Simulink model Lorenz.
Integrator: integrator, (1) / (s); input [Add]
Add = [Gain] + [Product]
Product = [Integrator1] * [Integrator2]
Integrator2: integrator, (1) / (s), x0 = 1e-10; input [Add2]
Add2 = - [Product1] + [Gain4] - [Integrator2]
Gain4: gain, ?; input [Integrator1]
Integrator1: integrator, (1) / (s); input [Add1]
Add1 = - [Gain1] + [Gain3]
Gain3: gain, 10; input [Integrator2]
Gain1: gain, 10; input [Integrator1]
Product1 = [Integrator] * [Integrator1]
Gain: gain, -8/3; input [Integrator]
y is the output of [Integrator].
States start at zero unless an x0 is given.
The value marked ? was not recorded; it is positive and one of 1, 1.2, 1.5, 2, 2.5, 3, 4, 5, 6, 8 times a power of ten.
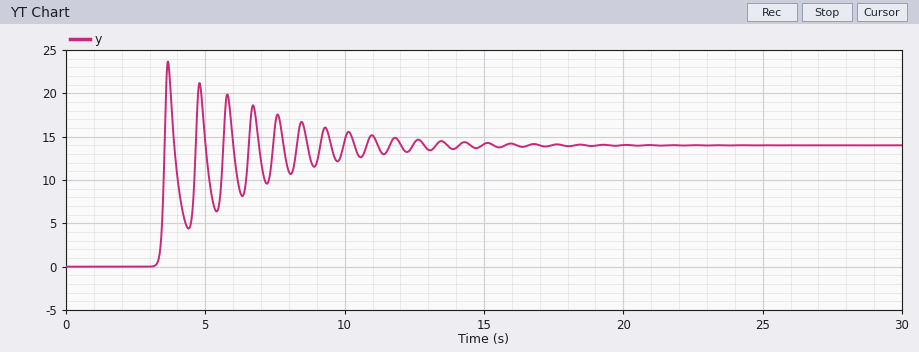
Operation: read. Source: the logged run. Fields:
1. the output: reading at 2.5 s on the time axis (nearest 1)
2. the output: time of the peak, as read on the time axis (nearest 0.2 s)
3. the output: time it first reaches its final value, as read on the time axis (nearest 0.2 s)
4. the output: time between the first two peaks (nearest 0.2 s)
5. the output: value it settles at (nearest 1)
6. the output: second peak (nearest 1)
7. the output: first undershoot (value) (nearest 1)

0
3.6 s
3.6 s
1.2 s
14
21
4
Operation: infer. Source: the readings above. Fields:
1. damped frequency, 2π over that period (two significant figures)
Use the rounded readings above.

5.2 rad/s
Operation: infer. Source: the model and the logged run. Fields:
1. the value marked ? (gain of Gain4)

15
